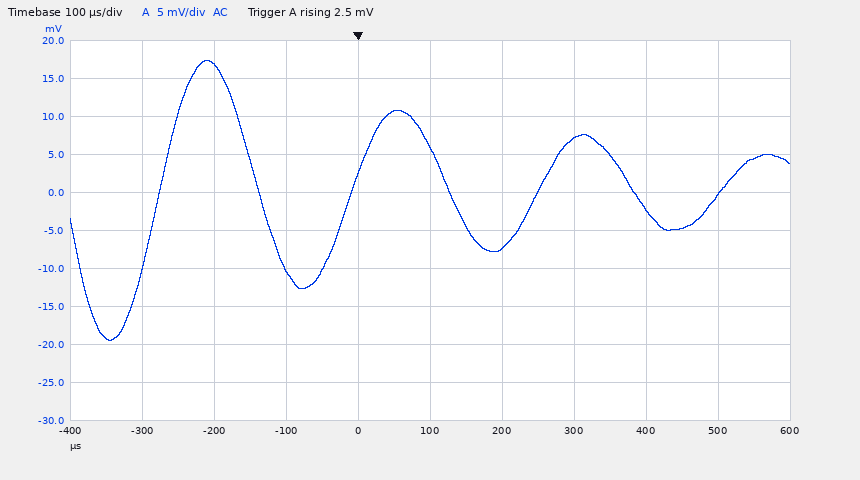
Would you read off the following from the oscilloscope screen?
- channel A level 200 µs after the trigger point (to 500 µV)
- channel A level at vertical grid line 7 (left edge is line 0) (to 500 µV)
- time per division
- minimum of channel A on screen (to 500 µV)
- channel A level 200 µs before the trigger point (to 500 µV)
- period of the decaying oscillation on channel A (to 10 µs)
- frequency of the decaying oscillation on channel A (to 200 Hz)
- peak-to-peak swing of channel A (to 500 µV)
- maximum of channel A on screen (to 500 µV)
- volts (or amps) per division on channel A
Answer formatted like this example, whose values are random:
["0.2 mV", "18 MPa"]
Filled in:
["-7.5 mV", "7.0 mV", "100 µs", "-19.5 mV", "17.0 mV", "260 µs", "3.8 kHz", "37.0 mV", "17.5 mV", "5 mV"]
